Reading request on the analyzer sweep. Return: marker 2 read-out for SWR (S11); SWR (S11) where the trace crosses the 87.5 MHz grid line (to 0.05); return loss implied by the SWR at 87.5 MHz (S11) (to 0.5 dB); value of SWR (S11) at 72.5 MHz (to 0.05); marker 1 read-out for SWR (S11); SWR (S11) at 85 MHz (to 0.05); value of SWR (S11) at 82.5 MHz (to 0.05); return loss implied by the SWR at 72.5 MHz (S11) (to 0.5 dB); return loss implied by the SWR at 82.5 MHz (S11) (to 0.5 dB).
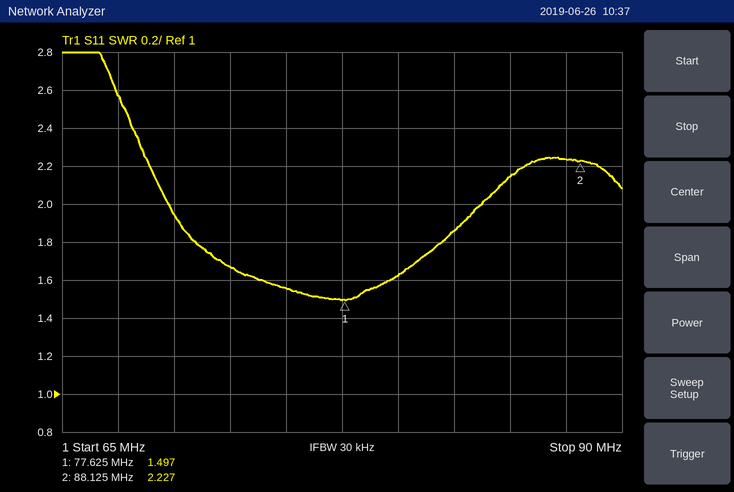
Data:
2.227
2.25
8.5 dB
1.65
1.497
2.15
1.85
12.0 dB
10.5 dB
